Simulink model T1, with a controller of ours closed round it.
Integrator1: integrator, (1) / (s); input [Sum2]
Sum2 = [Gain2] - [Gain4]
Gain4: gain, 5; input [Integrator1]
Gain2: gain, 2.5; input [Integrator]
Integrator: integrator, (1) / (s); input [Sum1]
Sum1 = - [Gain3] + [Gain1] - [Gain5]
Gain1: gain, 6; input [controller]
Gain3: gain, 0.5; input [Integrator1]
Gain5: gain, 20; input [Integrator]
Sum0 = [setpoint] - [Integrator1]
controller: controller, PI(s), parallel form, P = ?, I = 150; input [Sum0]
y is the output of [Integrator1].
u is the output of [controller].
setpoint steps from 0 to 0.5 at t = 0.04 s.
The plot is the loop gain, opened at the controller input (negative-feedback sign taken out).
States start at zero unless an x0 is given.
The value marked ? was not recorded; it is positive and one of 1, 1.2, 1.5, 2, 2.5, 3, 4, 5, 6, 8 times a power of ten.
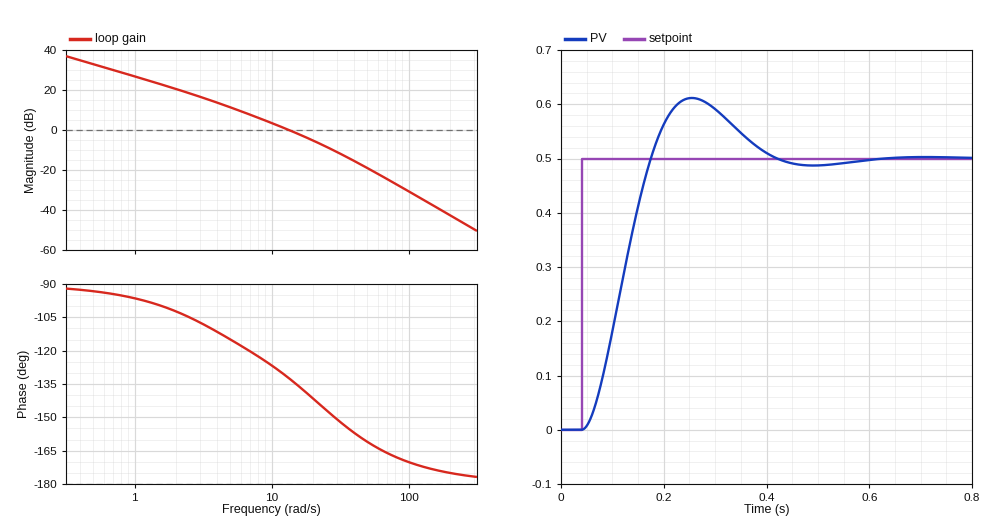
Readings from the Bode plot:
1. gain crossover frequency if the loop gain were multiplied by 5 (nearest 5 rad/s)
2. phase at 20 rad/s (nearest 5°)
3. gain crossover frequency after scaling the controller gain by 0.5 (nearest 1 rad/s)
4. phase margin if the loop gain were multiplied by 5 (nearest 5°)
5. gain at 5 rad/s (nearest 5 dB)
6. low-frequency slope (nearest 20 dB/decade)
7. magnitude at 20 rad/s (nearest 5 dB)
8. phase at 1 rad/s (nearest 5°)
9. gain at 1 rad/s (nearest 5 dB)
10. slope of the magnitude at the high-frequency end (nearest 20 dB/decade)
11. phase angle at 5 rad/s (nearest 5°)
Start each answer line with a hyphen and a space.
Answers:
- 35 rad/s
- -140°
- 8 rad/s
- 25°
- 10 dB
- -20 dB/decade
- -5 dB
- -95°
- 25 dB
- -40 dB/decade
- -115°
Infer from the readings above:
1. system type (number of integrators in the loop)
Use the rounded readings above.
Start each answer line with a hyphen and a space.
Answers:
- 1
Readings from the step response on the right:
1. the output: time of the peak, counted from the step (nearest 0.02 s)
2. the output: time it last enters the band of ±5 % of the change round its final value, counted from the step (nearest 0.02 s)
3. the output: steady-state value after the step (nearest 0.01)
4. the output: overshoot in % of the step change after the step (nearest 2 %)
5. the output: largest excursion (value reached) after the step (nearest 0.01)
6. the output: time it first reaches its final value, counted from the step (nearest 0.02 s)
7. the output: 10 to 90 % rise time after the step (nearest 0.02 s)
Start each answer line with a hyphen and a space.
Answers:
- 0.22 s
- 0.34 s
- 0.50
- 22 %
- 0.61
- 0.14 s
- 0.10 s
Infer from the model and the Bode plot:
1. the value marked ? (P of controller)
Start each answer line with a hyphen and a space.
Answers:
- 20
